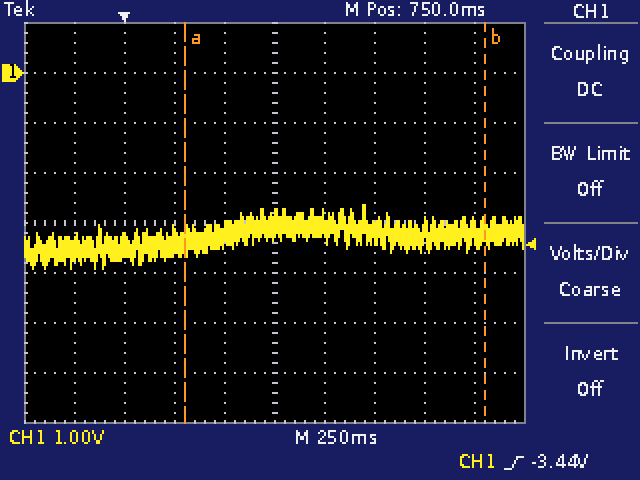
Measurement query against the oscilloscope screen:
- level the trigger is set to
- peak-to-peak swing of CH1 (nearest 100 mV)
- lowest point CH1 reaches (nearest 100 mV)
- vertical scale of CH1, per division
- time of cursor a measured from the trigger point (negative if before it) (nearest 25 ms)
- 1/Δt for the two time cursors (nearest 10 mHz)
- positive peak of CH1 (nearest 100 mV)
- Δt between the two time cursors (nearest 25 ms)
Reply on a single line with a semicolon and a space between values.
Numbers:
-3.44 V; 1.3 V; -3.9 V; 1 V; +300 ms; 670 mHz; -2.6 V; 1.500 s
